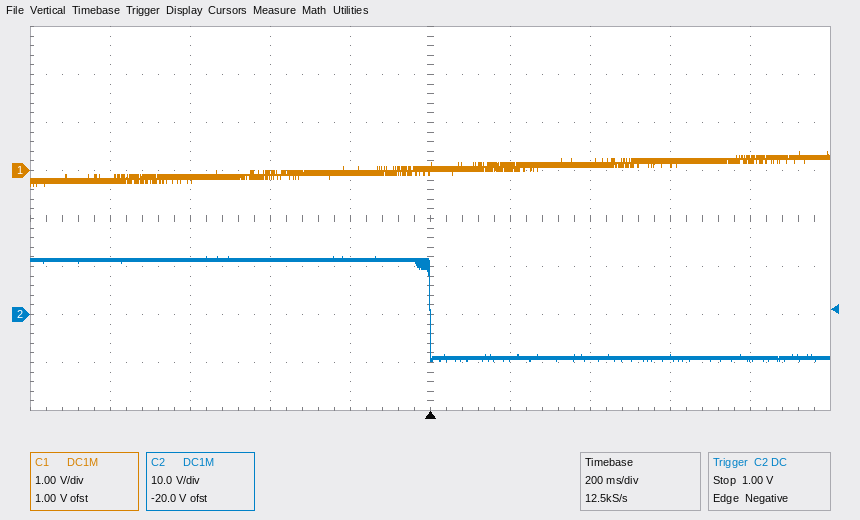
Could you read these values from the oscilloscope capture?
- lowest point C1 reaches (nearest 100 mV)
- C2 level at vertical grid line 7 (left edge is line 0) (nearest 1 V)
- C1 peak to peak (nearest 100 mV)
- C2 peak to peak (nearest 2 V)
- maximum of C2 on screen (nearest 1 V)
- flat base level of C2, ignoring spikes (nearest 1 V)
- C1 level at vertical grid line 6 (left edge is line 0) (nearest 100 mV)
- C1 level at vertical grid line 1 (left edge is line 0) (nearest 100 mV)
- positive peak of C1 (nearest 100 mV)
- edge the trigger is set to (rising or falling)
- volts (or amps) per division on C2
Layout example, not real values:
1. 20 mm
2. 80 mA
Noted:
1. -300 mV
2. -9 V
3. 700 mV
4. 22 V
5. 12 V
6. -9 V
7. 100 mV
8. -200 mV
9. 400 mV
10. falling
11. 10 V
